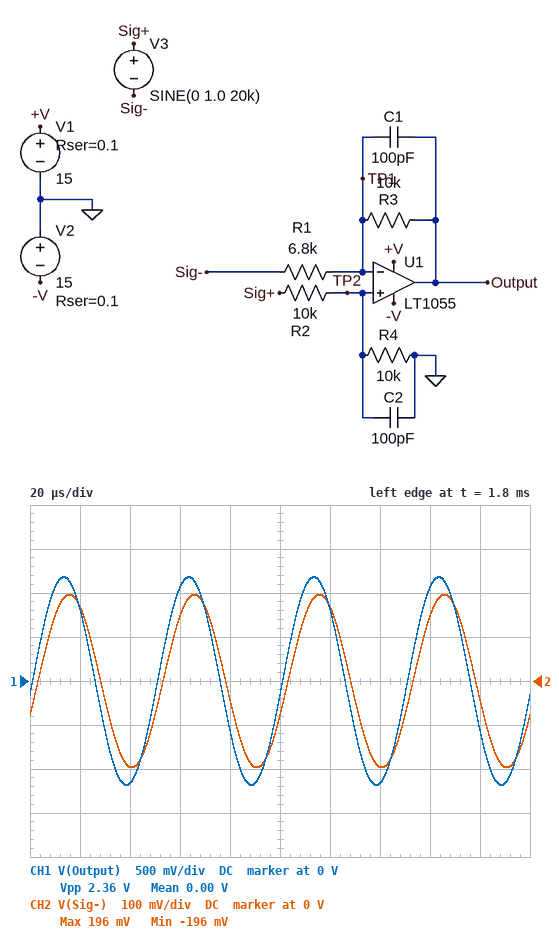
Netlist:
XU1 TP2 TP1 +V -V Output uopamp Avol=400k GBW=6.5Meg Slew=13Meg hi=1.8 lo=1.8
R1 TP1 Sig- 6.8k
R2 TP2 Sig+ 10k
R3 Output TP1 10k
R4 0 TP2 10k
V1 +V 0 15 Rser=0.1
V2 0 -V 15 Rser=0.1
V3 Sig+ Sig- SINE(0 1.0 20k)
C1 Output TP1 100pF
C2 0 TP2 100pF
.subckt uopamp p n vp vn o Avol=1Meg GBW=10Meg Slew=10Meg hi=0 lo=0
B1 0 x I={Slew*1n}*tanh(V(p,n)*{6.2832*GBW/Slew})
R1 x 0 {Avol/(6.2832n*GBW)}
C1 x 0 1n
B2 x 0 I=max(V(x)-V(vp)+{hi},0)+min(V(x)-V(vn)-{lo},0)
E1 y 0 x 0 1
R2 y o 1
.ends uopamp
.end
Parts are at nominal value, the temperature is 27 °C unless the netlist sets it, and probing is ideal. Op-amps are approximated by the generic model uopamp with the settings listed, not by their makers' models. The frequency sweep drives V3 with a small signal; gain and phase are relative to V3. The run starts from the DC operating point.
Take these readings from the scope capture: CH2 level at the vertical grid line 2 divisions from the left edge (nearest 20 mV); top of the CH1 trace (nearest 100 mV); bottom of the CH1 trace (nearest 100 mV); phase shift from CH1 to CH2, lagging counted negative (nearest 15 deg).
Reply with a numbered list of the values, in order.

1. -200 mV
2. 1.2 V
3. -1.2 V
4. -15 deg
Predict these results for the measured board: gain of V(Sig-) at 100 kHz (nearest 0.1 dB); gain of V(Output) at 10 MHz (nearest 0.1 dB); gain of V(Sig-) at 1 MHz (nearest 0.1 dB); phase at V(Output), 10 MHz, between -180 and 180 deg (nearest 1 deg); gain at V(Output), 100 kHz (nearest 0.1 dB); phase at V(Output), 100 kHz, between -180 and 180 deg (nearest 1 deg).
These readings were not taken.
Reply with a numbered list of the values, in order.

1. -11.1 dB
2. -39.8 dB
3. -7.6 dB
4. -145 deg
5. 0 dB
6. -34 deg
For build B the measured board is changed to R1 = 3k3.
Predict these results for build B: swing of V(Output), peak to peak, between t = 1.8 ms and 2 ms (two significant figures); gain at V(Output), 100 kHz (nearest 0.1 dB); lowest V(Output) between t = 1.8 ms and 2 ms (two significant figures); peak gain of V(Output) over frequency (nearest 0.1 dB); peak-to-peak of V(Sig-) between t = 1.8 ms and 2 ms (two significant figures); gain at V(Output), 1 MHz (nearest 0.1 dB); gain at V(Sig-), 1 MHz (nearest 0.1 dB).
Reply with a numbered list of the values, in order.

1. 3.0 V
2. 2.0 dB
3. -1.5 V
4. 3.5 dB
5. 1.0 V
6. -12.9 dB
7. -11.1 dB
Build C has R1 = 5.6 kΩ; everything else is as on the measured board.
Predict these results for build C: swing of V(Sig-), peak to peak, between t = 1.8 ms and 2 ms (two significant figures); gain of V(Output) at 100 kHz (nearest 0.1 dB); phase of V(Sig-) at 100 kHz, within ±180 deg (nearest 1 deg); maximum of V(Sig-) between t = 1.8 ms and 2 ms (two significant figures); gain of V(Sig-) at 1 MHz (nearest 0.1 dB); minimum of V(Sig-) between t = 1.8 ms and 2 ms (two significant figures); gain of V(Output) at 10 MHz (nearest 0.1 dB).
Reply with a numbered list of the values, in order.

1. 570 mV
2. 0.6 dB
3. -74 deg
4. 280 mV
5. -8.5 dB
6. -280 mV
7. -39.1 dB
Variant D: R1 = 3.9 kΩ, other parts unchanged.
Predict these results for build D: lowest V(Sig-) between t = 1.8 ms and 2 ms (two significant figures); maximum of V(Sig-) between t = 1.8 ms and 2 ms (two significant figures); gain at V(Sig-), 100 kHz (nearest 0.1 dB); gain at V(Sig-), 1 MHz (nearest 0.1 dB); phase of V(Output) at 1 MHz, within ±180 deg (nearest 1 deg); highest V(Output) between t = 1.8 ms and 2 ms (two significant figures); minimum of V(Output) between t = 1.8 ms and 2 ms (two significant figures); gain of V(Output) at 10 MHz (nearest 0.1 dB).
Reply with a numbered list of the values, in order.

1. -440 mV
2. 440 mV
3. -7.9 dB
4. -10.3 dB
5. -90 deg
6. 1.4 V
7. -1.4 V
8. -38.1 dB
